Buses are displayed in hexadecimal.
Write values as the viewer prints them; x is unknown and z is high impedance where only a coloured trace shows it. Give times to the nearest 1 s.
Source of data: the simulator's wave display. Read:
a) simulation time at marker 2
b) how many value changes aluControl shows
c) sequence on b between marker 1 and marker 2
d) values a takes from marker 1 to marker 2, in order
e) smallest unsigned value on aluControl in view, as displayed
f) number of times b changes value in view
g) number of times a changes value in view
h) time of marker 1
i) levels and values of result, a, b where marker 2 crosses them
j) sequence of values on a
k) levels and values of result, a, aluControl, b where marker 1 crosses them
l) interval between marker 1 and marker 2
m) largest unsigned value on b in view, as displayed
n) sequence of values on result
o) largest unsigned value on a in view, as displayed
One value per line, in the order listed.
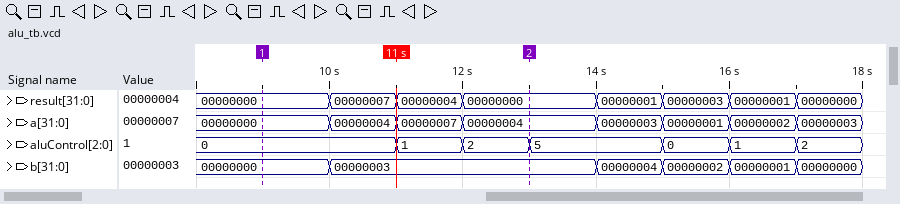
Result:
13 s
6
00000000, 00000003
00000000, 00000004, 00000007, 00000004
0
5
7
9 s
result=00000000, a=00000004, b=00000003
00000000, 00000004, 00000007, 00000004, 00000003, 00000001, 00000002, 00000003
result=00000000, a=00000000, aluControl=0, b=00000000
4 s
00000004
00000000, 00000007, 00000004, 00000000, 00000001, 00000003, 00000001, 00000000
00000007
